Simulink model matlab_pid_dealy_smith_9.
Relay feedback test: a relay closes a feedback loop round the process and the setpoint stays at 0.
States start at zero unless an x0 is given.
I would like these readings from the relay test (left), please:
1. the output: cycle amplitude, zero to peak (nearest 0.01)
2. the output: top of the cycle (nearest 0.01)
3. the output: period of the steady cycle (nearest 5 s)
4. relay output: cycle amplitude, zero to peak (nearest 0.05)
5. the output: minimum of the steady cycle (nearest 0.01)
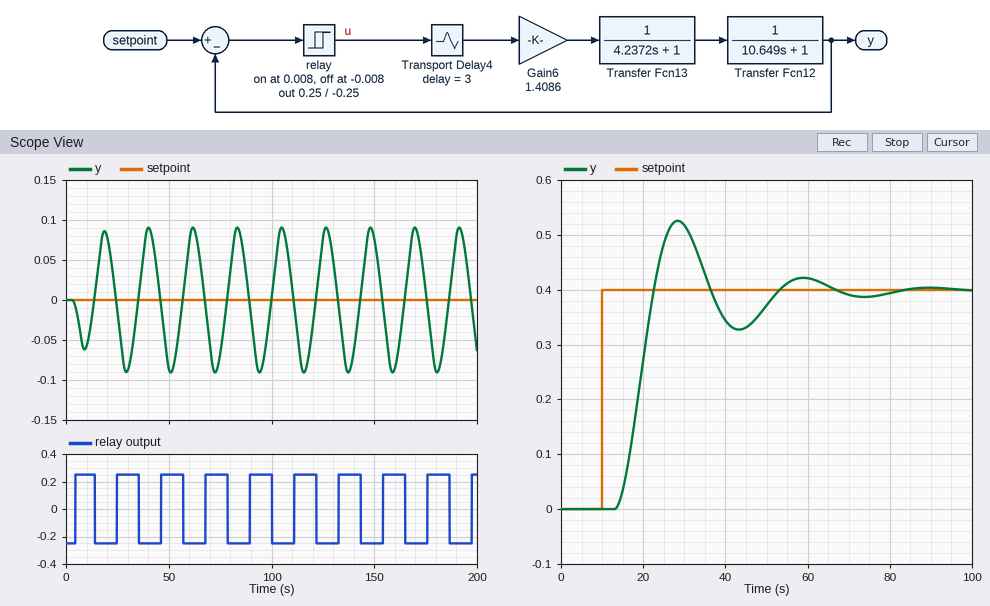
0.09
0.09
20 s
0.25
-0.09
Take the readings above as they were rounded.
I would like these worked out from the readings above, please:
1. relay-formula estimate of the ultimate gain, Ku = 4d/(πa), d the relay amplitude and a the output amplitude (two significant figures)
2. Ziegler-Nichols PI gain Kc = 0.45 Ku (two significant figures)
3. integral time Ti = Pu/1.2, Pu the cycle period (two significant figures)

3.5
1.6
17 s
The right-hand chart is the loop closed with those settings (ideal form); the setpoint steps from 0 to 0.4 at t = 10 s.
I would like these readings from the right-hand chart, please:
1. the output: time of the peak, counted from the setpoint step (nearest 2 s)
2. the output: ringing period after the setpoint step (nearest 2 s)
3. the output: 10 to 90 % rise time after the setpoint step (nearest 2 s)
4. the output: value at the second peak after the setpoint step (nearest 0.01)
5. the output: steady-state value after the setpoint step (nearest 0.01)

18 s
30 s
6 s
0.42
0.40
